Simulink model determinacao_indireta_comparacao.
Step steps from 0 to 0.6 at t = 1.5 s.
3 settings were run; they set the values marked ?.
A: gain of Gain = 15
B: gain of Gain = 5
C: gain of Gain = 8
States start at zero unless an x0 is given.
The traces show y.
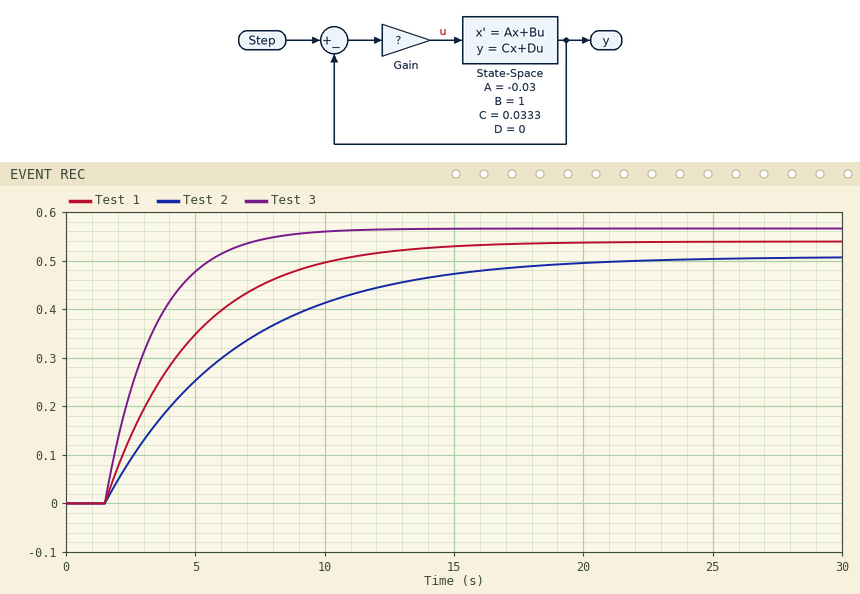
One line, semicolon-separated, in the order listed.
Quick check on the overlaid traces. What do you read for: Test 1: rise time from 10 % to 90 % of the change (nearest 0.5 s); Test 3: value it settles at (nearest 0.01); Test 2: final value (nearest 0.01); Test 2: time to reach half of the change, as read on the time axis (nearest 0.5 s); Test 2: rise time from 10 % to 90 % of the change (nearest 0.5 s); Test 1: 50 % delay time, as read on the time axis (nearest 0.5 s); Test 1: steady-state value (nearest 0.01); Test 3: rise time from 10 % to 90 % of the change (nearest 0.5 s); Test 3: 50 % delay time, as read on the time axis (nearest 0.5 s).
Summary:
7.5 s; 0.57; 0.51; 5.0 s; 11.0 s; 4.0 s; 0.54; 4.0 s; 3.0 s
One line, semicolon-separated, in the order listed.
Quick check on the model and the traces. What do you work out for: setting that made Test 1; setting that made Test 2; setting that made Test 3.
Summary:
C; B; A
